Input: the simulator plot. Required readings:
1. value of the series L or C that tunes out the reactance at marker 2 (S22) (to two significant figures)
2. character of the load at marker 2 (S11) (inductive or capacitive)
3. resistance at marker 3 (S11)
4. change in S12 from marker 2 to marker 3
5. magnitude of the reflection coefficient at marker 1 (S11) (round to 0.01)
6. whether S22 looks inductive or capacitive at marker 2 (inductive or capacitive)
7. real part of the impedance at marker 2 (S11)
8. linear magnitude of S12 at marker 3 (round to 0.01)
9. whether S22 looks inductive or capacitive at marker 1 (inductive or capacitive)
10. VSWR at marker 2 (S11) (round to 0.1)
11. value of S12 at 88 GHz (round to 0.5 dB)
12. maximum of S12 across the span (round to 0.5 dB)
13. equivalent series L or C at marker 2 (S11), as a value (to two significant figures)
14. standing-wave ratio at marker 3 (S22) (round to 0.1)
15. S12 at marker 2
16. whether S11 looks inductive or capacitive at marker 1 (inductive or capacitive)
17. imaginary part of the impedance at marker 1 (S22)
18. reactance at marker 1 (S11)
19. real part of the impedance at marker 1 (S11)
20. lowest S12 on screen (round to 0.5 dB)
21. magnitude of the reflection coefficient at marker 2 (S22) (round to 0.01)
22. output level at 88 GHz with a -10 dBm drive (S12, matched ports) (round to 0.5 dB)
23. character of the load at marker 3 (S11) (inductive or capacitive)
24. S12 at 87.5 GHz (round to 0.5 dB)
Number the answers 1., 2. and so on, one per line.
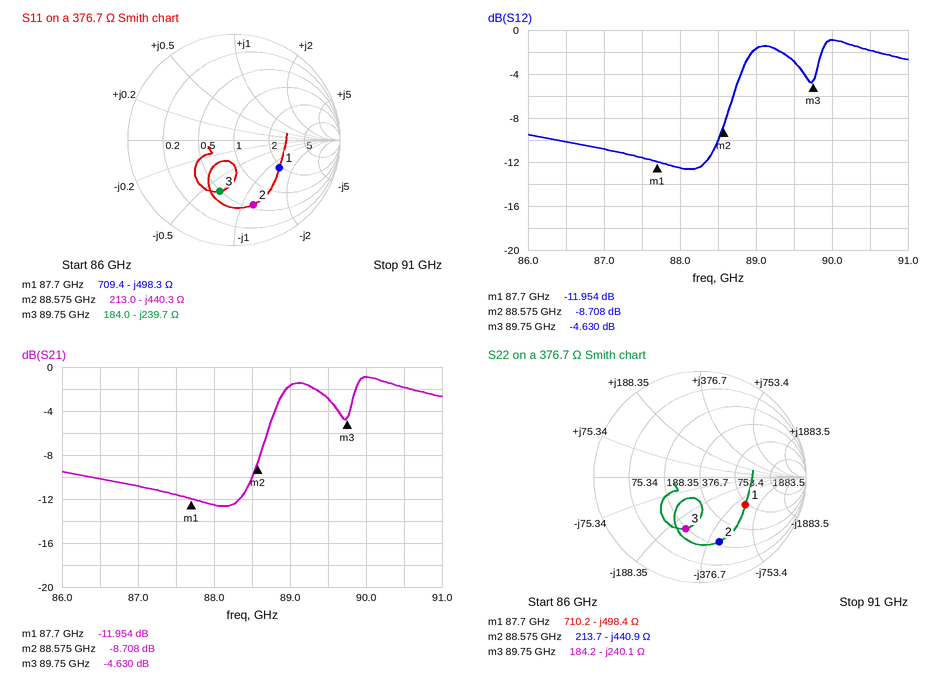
1. 790 pH
2. capacitive
3. 184.0 Ω
4. 4.078 dB
5. 0.50
6. capacitive
7. 213.0 Ω
8. 0.59
9. capacitive
10. 4.5
11. -12.5 dB
12. -1.0 dB
13. 4.1 fF
14. 3.0
15. -8.708 dB
16. capacitive
17. -498.4 Ω
18. -498.3 Ω
19. 709.4 Ω
20. -12.5 dB
21. 0.64
22. -22.5 dBm
23. capacitive
24. -11.5 dB
